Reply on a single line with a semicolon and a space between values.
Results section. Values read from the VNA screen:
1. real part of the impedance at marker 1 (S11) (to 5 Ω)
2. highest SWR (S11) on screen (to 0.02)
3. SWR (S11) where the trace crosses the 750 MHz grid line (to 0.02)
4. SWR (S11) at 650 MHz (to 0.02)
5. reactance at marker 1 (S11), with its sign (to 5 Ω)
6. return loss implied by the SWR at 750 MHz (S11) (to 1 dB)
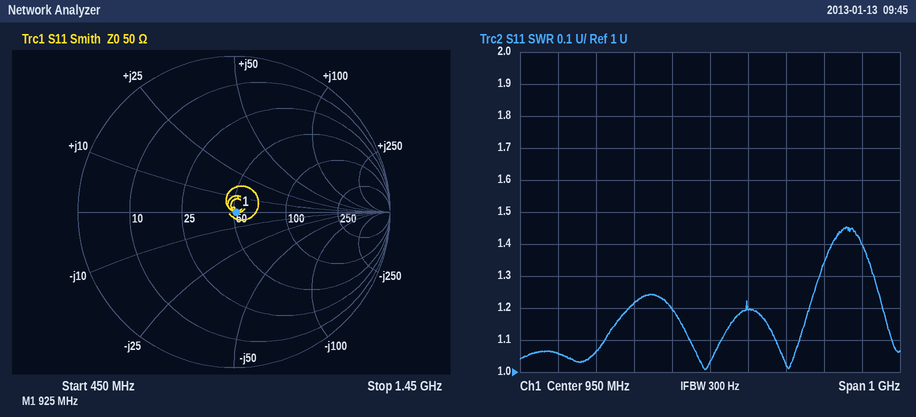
50 Ω; 1.46; 1.22; 1.06; 0 Ω; 20 dB
